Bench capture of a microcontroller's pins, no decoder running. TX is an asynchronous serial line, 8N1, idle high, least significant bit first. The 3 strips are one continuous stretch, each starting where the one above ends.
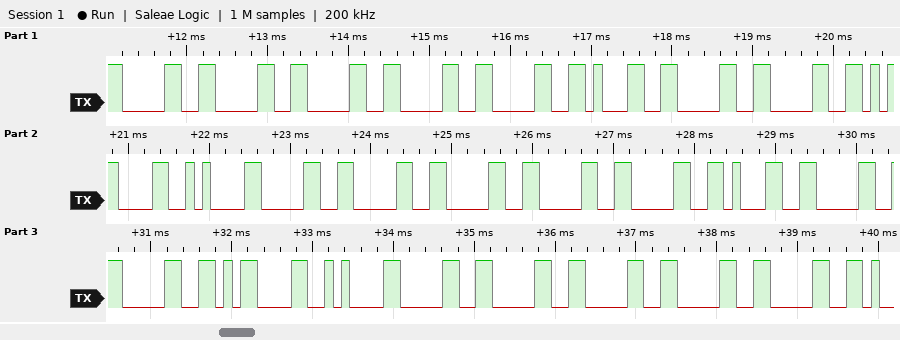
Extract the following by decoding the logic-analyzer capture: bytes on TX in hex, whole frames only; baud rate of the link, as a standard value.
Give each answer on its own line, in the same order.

0x30 0x30 0x30 0x30 0x30 0x31 0x30 0x30 0x0D 0x0A 0x30 0x30 0x30 0x30 0x30 0x31 0x30 0x30 0x0D 0x0A 0x30 0x30 0x30 0x30 0x30
9600 baud
